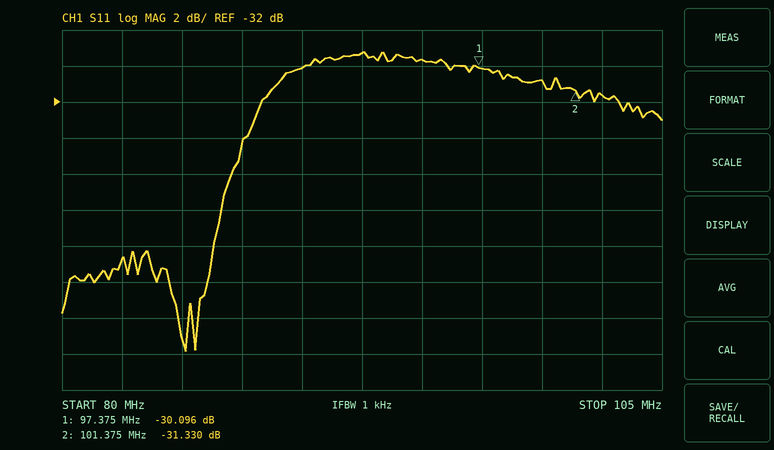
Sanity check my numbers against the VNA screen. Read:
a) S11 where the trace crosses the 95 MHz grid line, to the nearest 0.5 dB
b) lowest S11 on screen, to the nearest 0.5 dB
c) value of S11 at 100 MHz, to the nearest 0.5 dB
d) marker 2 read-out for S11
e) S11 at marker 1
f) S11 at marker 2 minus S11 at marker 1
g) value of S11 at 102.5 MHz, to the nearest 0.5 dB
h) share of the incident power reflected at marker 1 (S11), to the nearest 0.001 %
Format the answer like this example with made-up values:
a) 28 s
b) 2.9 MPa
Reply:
a) -29.5 dB
b) -46.0 dB
c) -31.0 dB
d) -31.330 dB
e) -30.096 dB
f) -1.234 dB
g) -31.5 dB
h) 0.098 %
